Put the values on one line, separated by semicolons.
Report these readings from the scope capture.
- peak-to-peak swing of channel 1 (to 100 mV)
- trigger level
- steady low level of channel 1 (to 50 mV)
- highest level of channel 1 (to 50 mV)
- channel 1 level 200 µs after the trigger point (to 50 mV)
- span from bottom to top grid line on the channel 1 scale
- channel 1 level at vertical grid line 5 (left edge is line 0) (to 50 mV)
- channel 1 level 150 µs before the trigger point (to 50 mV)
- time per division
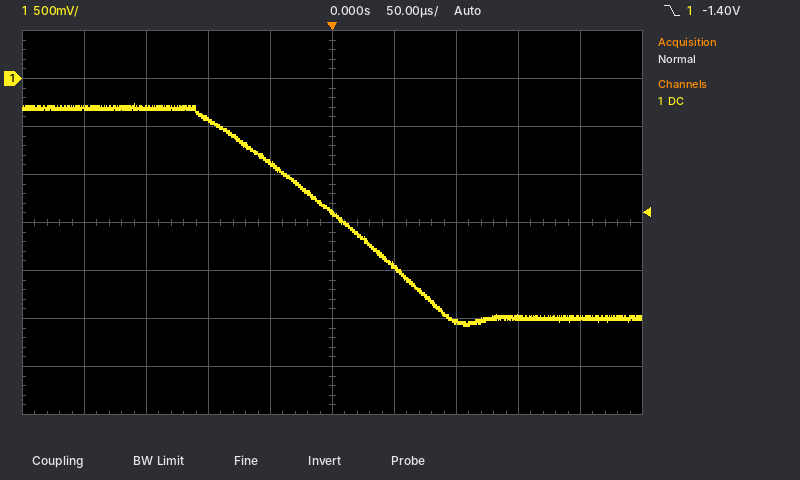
2.30 V; -1.40 V; -2.50 V; -250 mV; -2.50 V; 4 V; -1.40 V; -300 mV; 50 µs
